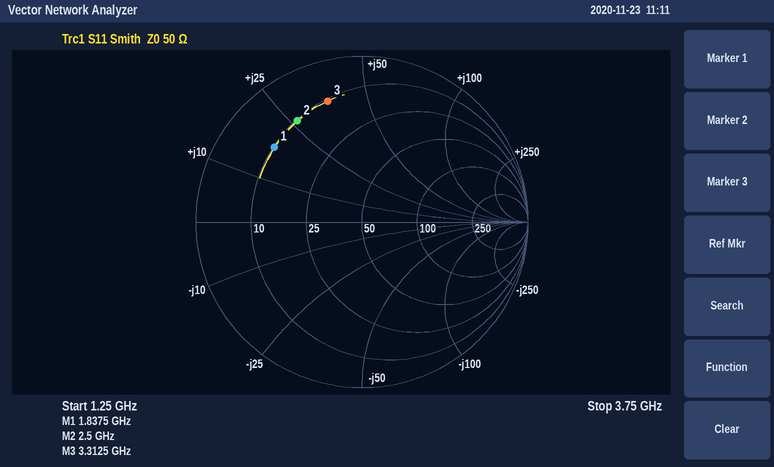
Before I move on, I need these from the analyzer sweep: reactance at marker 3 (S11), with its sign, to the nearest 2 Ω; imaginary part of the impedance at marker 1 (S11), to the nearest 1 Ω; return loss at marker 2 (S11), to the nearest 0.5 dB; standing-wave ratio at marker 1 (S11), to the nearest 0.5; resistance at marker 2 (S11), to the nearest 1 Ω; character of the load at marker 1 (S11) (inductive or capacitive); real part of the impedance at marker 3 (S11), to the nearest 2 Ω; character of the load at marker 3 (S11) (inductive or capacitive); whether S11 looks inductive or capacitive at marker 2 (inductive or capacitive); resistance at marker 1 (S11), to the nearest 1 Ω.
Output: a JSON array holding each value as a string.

["+36 Ω", "+18 Ω", "3.0 dB", "5.5", "10 Ω", "inductive", "10 Ω", "inductive", "inductive", "10 Ω"]
